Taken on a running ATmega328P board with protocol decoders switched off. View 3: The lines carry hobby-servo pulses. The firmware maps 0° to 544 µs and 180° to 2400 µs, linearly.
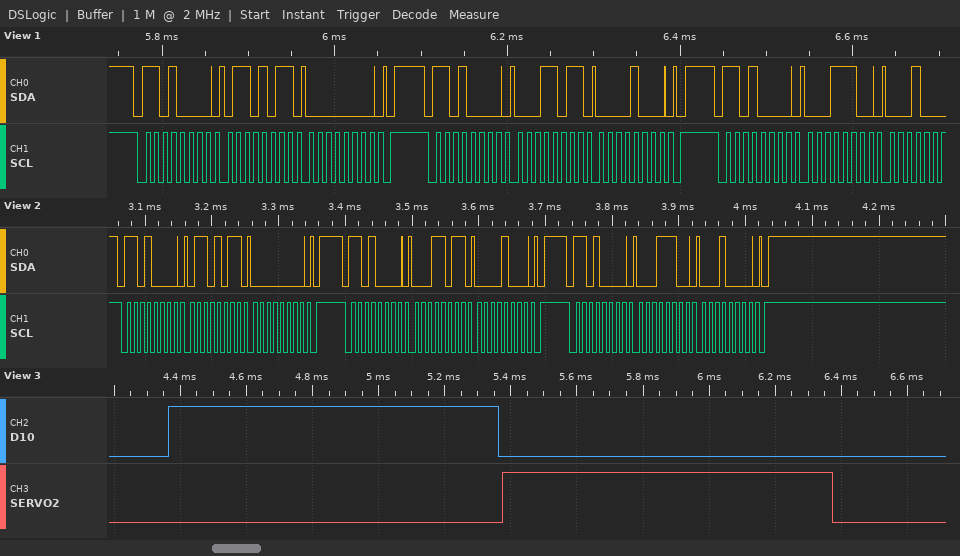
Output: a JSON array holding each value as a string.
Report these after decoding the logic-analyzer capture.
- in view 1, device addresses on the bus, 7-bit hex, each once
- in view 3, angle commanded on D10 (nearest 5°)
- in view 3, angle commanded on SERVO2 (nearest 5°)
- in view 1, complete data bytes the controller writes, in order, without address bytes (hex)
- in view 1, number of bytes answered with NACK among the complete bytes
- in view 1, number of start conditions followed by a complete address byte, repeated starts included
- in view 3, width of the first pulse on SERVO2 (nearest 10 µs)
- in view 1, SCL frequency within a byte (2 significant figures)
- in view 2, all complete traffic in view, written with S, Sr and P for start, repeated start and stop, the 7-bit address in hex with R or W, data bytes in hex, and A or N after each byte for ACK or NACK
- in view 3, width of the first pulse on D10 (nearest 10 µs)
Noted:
["0x68", "45°", "45°", "6B 00 1B 08 1C", "0", "3", "1000 µs", "100 kHz", "S 68W A 6B A 00 A P S 68W A 1B A 08 A P S 68W A 1C A 10 A P", "1000 µs"]
